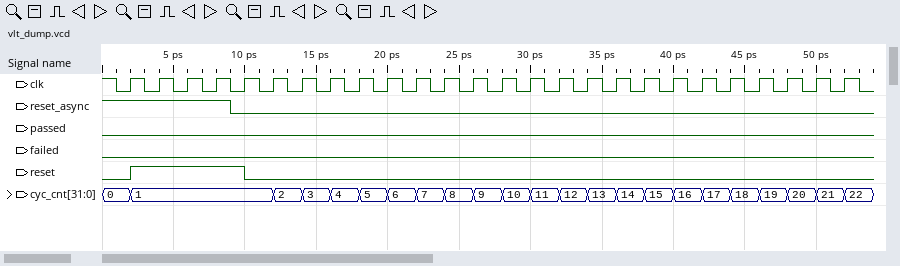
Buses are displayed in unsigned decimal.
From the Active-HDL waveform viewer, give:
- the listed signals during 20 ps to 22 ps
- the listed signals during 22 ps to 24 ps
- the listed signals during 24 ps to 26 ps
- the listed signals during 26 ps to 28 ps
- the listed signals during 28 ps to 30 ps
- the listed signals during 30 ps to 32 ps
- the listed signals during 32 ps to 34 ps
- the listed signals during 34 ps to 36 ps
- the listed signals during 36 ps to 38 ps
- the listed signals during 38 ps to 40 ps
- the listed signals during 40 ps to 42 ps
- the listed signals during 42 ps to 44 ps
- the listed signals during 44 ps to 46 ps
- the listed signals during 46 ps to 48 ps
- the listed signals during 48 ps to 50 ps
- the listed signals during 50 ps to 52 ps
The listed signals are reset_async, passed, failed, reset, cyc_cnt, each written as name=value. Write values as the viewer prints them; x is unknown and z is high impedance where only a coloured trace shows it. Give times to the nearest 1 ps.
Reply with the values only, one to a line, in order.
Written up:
reset_async=0, passed=0, failed=0, reset=0, cyc_cnt=6
reset_async=0, passed=0, failed=0, reset=0, cyc_cnt=7
reset_async=0, passed=0, failed=0, reset=0, cyc_cnt=8
reset_async=0, passed=0, failed=0, reset=0, cyc_cnt=9
reset_async=0, passed=0, failed=0, reset=0, cyc_cnt=10
reset_async=0, passed=0, failed=0, reset=0, cyc_cnt=11
reset_async=0, passed=0, failed=0, reset=0, cyc_cnt=12
reset_async=0, passed=0, failed=0, reset=0, cyc_cnt=13
reset_async=0, passed=0, failed=0, reset=0, cyc_cnt=14
reset_async=0, passed=0, failed=0, reset=0, cyc_cnt=15
reset_async=0, passed=0, failed=0, reset=0, cyc_cnt=16
reset_async=0, passed=0, failed=0, reset=0, cyc_cnt=17
reset_async=0, passed=0, failed=0, reset=0, cyc_cnt=18
reset_async=0, passed=0, failed=0, reset=0, cyc_cnt=19
reset_async=0, passed=0, failed=0, reset=0, cyc_cnt=20
reset_async=0, passed=0, failed=0, reset=0, cyc_cnt=21
